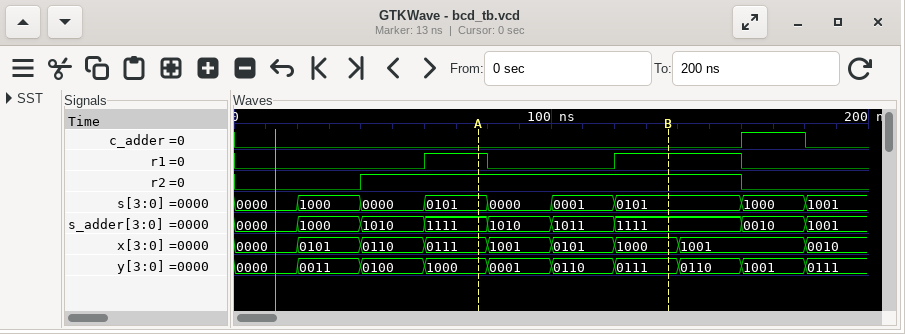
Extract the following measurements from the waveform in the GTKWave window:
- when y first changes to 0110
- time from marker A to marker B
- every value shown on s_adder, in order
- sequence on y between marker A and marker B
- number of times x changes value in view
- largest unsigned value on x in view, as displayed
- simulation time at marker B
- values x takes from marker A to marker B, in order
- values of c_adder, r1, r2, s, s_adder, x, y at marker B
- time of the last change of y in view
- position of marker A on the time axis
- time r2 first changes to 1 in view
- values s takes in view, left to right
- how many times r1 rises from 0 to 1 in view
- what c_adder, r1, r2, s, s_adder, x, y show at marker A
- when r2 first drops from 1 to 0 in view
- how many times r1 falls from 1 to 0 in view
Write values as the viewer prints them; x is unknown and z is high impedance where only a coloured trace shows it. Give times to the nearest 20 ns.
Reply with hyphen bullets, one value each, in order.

- 100 ns
- 60 ns
- 0000, 1000, 1010, 1111, 1010, 1011, 1111, 0010, 1001
- 1000, 0001, 0110, 0111
- 8
- 1001
- 140 ns
- 0111, 1001, 0101, 1000
- c_adder=0, r1=1, r2=1, s=0101, s_adder=1111, x=1000, y=0111
- 180 ns
- 80 ns
- 40 ns
- 0000, 1000, 0000, 0101, 0000, 0001, 0101, 1000, 1001
- 2
- c_adder=0, r1=1, r2=1, s=0101, s_adder=1111, x=0111, y=1000
- 160 ns
- 2
